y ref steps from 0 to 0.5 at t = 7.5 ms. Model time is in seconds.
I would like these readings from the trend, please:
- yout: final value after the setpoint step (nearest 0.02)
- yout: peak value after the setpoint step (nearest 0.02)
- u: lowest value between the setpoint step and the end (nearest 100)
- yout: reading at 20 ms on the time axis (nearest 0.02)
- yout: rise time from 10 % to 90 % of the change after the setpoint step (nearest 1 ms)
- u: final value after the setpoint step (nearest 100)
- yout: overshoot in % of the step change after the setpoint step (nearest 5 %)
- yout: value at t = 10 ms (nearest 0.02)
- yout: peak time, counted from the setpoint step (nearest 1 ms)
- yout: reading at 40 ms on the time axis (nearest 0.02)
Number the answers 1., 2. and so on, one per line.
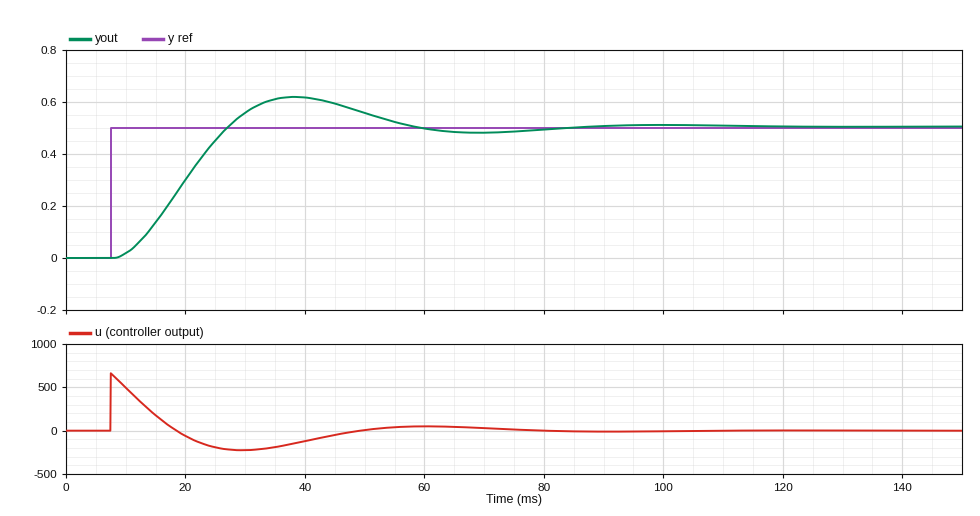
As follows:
1. 0.50
2. 0.62
3. -200
4. 0.30
5. 13 ms
6. 0
7. 25 %
8. 0.02
9. 31 ms
10. 0.62
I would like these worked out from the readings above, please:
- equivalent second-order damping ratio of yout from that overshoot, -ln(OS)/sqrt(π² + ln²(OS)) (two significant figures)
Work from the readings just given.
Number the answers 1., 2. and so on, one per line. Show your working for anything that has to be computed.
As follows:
1. ln(0.25) = -1.386; 1.386 / sqrt(9.870 + 1.922) = 0.40
